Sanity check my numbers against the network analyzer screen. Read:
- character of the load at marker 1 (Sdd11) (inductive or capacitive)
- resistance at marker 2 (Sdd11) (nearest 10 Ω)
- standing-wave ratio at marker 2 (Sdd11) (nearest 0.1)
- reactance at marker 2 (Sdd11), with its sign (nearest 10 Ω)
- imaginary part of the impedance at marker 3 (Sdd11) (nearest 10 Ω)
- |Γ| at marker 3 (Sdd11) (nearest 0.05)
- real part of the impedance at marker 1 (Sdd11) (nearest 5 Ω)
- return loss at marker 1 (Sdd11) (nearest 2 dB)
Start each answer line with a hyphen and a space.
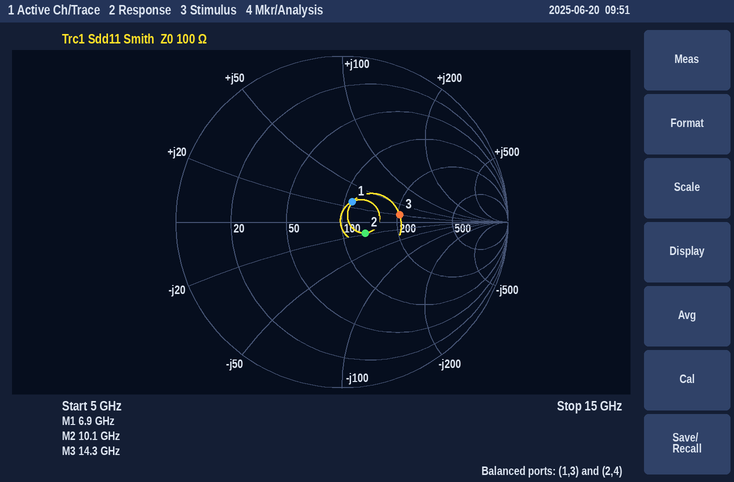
- inductive
- 130 Ω
- 1.4
- -20 Ω
- +20 Ω
- 0.35
- 110 Ω
- 18 dB
